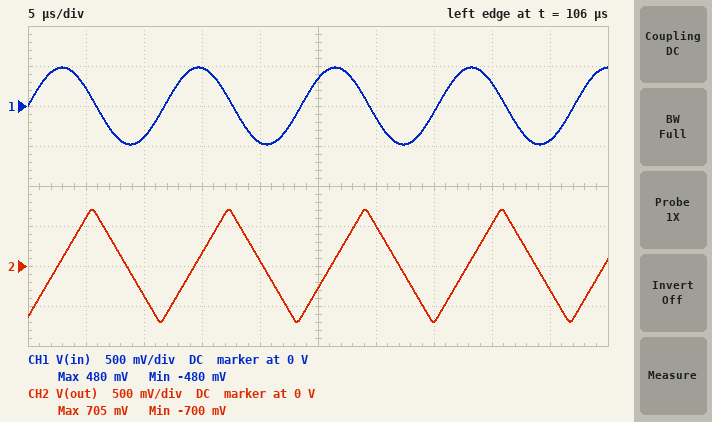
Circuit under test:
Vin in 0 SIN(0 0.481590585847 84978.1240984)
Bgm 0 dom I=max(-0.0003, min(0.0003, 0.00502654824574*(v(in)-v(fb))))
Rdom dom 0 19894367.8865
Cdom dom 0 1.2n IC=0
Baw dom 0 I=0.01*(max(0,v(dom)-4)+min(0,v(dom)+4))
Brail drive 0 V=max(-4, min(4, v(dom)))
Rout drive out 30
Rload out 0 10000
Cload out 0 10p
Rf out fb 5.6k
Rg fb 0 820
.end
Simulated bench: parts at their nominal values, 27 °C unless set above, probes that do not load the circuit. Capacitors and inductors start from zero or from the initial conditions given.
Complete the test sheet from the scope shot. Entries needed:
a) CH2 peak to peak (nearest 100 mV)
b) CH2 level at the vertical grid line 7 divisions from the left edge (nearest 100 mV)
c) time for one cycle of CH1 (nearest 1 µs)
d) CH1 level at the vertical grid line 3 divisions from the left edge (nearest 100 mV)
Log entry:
1.4 V
-700 mV
12 µs
500 mV
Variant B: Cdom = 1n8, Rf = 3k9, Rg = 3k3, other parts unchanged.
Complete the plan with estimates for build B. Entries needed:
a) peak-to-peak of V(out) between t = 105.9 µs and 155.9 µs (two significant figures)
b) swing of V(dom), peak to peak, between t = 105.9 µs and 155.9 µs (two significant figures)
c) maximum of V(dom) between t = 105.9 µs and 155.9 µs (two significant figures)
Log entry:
930 mV
940 mV
470 mV
